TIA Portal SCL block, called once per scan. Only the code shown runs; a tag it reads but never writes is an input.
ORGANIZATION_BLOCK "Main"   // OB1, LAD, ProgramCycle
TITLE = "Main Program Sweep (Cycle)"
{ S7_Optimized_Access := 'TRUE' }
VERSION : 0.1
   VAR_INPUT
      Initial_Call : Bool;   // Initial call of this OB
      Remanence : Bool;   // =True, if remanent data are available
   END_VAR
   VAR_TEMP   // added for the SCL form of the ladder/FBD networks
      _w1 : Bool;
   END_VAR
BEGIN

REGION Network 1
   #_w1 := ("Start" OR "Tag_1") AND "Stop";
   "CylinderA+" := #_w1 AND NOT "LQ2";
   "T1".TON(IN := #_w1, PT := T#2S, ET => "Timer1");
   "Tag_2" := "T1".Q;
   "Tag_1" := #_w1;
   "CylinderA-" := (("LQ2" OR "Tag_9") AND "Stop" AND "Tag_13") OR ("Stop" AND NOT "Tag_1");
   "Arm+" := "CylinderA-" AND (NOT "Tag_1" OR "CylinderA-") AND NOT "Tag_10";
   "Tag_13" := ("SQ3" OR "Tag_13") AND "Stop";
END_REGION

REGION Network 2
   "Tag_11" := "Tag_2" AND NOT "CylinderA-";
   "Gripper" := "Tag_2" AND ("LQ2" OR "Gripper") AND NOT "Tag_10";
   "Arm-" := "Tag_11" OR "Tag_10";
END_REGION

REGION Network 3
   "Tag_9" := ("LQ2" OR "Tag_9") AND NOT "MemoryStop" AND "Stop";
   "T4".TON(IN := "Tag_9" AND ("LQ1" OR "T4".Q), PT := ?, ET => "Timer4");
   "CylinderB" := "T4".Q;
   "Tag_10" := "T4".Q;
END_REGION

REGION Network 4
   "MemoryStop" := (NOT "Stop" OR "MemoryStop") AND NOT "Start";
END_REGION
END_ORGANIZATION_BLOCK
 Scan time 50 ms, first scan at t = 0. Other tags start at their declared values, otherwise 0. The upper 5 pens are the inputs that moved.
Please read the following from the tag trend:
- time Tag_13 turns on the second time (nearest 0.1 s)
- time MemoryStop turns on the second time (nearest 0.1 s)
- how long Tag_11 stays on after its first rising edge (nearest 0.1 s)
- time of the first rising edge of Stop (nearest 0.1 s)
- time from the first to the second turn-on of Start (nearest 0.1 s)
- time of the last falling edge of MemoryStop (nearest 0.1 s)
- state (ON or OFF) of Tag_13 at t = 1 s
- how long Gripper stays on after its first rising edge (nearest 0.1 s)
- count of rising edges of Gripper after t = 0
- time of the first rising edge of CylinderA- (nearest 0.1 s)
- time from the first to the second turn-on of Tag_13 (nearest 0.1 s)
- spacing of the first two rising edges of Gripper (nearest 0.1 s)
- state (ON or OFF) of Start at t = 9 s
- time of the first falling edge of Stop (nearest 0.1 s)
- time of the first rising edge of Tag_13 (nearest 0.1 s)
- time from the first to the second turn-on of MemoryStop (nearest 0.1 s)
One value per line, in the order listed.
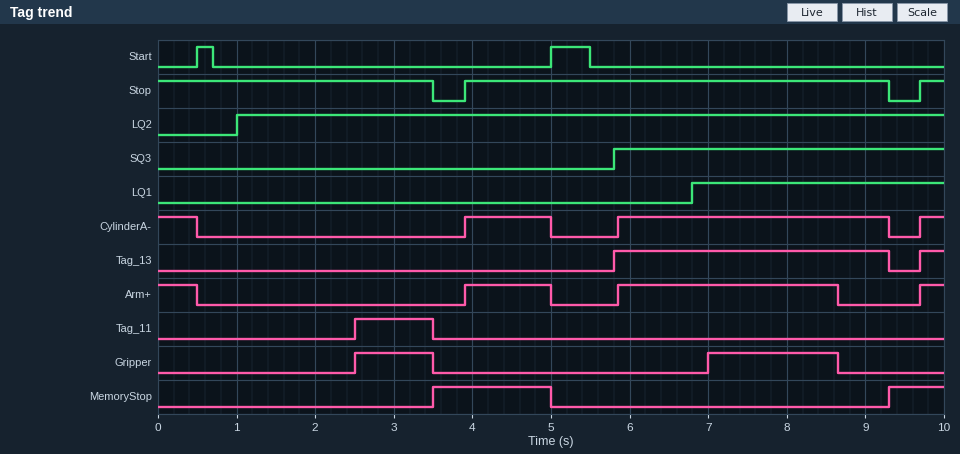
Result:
9.7 s
9.3 s
1.0 s
3.9 s
4.5 s
5.0 s
OFF
1.0 s
2
3.9 s
3.9 s
4.5 s
OFF
3.5 s
5.8 s
5.8 s
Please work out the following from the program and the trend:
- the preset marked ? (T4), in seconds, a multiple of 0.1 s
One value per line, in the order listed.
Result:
1.8 s
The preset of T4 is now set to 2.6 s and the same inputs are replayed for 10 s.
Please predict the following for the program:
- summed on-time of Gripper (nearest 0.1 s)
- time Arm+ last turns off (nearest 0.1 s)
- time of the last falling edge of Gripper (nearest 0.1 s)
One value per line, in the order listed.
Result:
3.3 s
9.3 s
9.3 s
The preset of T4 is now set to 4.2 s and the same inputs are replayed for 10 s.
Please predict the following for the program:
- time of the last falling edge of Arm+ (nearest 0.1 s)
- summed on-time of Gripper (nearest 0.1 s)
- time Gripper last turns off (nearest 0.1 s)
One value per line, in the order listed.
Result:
9.3 s
3.3 s
9.3 s
